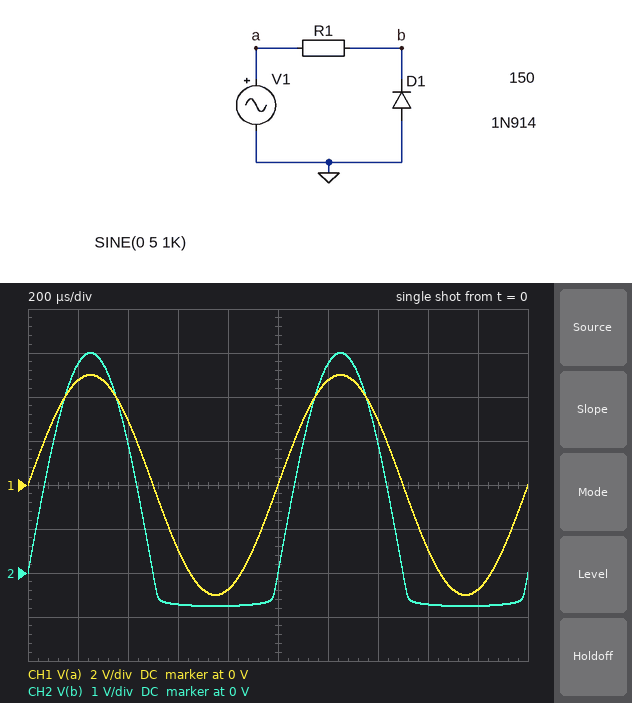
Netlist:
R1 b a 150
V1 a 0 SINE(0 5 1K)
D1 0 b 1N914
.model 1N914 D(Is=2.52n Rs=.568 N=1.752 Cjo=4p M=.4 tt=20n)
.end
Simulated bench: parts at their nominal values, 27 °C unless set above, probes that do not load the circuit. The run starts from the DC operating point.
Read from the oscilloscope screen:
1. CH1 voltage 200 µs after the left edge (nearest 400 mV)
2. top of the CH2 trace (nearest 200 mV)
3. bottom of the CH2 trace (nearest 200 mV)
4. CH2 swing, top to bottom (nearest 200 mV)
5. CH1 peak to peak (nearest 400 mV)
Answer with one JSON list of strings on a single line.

["4.8 V", "5.0 V", "-800 mV", "5.8 V", "10.0 V"]
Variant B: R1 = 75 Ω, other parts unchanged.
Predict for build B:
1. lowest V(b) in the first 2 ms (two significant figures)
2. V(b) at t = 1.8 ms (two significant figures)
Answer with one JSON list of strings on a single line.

["-800 mV", "-790 mV"]
